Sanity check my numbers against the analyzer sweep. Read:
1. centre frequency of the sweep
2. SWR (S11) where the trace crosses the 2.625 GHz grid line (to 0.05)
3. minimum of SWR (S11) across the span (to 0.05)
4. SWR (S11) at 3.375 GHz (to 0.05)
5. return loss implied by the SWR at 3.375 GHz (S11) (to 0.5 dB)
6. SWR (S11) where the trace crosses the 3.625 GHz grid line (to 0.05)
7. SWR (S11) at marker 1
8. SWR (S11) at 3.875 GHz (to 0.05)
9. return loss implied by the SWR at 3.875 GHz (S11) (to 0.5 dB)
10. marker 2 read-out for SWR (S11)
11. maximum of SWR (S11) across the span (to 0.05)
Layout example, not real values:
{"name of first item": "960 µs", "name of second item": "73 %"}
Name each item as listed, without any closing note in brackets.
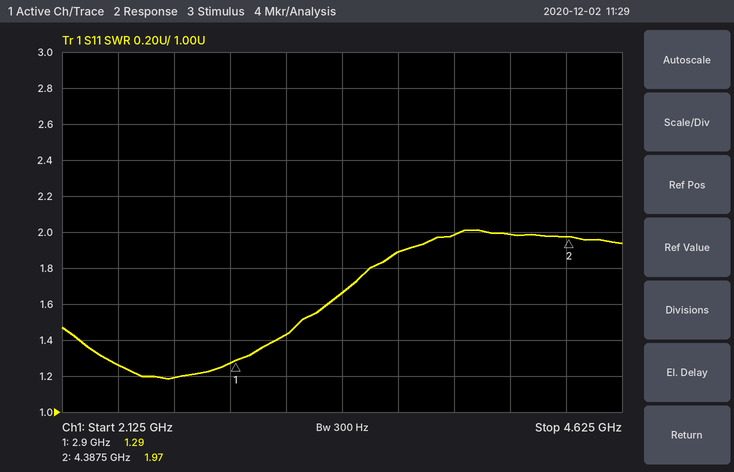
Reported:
{"centre frequency of the sweep": "3.375 GHz", "SWR (S11) where the trace crosses the 2.625 GHz grid line": "1.20", "minimum of SWR (S11) across the span": "1.20", "SWR (S11) at 3.375 GHz": "1.65", "return loss implied by the SWR at 3.375 GHz (S11)": "12.0 dB", "SWR (S11) where the trace crosses the 3.625 GHz grid line": "1.90", "SWR (S11) at marker 1": "1.29", "SWR (S11) at 3.875 GHz": "2.00", "return loss implied by the SWR at 3.875 GHz (S11)": "9.5 dB", "marker 2 read-out for SWR": "1.97", "maximum of SWR (S11) across the span": "2.00"}
